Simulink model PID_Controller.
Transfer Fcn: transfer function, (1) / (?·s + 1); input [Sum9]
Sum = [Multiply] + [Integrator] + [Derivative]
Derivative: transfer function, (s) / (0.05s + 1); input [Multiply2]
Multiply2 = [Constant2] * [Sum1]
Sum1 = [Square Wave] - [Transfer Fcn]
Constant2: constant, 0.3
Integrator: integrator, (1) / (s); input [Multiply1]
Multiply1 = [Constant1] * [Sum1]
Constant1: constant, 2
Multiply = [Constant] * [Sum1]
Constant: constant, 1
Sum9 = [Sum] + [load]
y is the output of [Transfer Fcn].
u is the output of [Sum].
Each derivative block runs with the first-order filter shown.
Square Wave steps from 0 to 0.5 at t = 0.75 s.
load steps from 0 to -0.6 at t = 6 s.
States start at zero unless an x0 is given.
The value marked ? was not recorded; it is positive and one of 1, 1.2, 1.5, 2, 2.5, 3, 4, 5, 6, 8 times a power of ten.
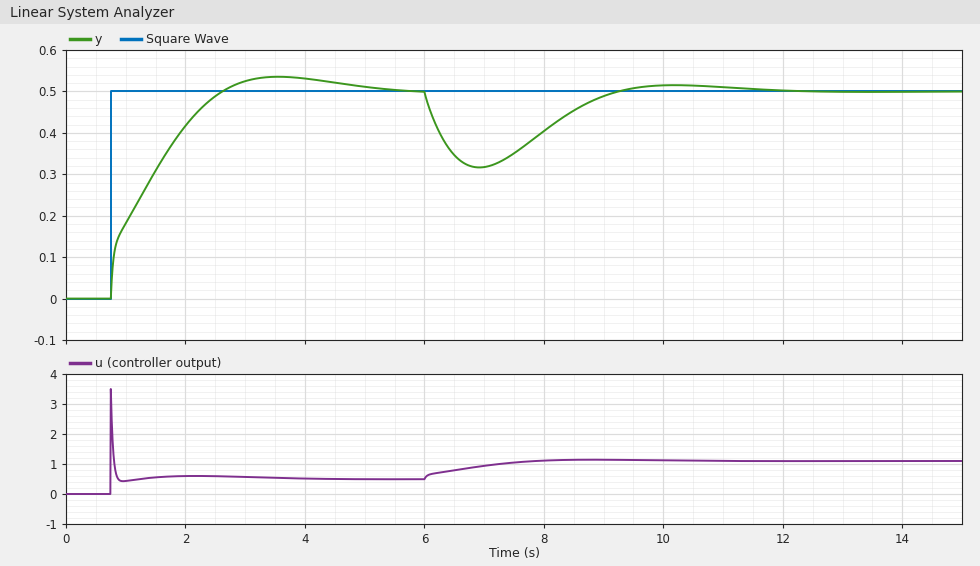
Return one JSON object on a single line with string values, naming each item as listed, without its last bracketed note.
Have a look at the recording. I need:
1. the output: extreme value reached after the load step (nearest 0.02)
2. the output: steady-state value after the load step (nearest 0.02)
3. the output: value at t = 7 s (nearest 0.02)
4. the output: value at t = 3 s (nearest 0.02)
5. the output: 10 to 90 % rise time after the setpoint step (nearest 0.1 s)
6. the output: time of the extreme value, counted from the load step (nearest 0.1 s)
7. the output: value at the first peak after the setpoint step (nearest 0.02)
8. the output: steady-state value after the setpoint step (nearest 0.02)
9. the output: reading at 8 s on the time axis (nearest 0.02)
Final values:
{"the output: extreme value reached after the load step": "0.32", "the output: steady-state value after the load step": "0.50", "the output: value at t = 7 s": "0.32", "the output: value at t = 3 s": "0.52", "the output: 10 to 90 % rise time after the setpoint step": "1.4 s", "the output: time of the extreme value, counted from the load step": "0.9 s", "the output: value at the first peak after the setpoint step": "0.54", "the output: steady-state value after the setpoint step": "0.50", "the output: reading at 8 s on the time axis": "0.40"}
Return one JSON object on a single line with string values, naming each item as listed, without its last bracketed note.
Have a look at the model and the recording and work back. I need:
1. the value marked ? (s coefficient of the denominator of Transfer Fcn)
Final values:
{"the value marked ?": "1"}
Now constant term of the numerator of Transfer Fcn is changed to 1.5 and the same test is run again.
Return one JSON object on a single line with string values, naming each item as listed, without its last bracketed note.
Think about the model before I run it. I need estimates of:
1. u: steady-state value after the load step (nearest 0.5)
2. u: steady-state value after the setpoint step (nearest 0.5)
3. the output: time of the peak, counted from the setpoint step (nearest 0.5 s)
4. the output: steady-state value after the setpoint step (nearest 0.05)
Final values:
{"u: steady-state value after the load step": "1.0", "u: steady-state value after the setpoint step": "0.5", "the output: time of the peak, counted from the setpoint step": "2.5 s", "the output: steady-state value after the setpoint step": "0.50"}
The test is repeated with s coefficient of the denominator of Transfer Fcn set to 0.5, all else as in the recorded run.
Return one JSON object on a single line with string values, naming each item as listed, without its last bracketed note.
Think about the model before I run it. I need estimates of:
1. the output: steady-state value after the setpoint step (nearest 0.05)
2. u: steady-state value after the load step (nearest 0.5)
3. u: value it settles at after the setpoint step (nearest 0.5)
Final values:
{"the output: steady-state value after the setpoint step": "0.50", "u: steady-state value after the load step": "1.0", "u: value it settles at after the setpoint step": "0.5"}
